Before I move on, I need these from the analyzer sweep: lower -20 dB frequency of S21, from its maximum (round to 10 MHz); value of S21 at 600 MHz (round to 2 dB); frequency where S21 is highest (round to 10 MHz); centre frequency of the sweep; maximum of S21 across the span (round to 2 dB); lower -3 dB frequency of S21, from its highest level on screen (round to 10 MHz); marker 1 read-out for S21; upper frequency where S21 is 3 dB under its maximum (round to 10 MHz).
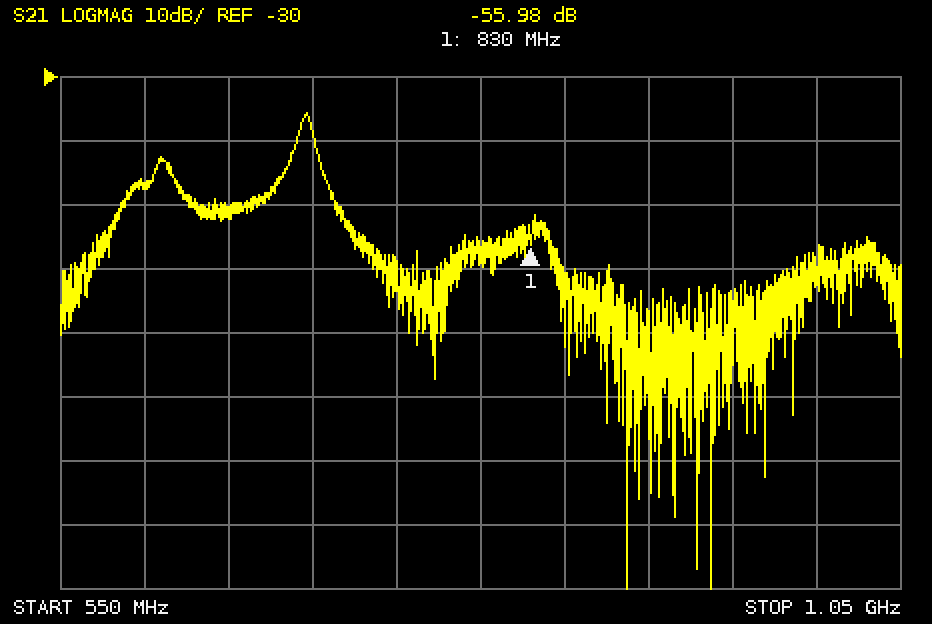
580 MHz
-48 dB
700 MHz
800 MHz
-36 dB
690 MHz
-55.98 dB
700 MHz
